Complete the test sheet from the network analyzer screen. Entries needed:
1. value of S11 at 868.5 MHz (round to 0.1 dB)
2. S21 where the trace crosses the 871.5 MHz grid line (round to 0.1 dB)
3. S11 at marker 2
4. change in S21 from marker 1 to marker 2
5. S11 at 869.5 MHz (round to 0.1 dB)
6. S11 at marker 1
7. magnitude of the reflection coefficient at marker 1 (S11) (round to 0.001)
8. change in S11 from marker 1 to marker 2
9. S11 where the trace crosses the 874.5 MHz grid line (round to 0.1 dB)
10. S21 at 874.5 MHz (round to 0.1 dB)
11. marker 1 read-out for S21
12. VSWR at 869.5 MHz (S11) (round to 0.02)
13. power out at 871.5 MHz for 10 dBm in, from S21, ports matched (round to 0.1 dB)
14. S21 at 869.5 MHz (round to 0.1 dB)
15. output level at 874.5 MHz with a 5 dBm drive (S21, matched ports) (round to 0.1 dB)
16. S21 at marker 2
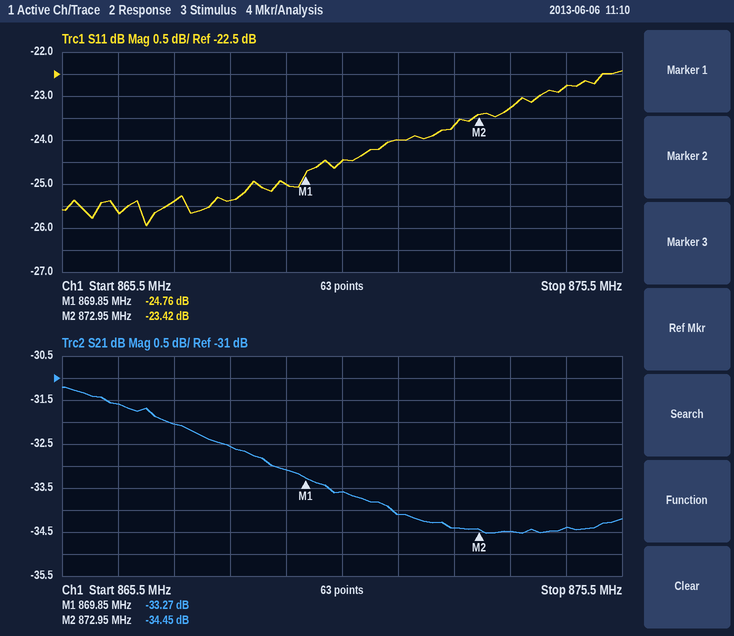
-25.4 dB
-34.1 dB
-23.42 dB
-1.18 dB
-25.0 dB
-24.76 dB
0.058
1.34 dB
-22.8 dB
-34.4 dB
-33.27 dB
1.12
-24.1 dBm
-33.1 dB
-29.4 dBm
-34.45 dB
